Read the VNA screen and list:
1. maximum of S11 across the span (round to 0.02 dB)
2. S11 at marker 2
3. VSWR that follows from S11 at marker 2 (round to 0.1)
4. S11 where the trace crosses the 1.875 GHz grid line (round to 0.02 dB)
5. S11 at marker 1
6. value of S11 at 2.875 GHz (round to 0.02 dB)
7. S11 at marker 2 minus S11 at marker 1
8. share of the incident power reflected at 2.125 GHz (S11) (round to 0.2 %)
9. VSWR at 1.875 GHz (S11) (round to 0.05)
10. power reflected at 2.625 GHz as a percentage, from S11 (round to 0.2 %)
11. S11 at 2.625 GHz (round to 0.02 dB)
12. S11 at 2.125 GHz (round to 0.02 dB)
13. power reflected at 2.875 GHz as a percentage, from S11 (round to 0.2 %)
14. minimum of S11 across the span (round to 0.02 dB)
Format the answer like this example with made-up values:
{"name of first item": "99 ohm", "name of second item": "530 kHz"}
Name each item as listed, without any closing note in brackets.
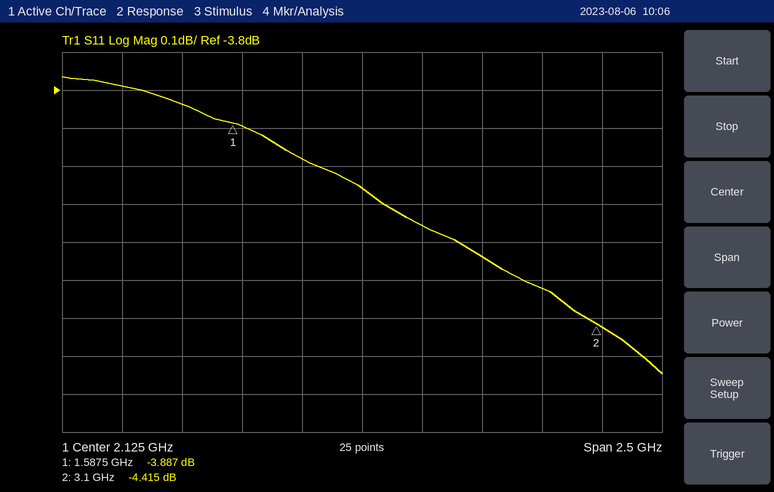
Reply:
{"maximum of S11 across the span": "-3.76 dB", "S11 at marker 2": "-4.415 dB", "VSWR that follows from S11 at marker 2": "4.0", "S11 where the trace crosses the 1.875 GHz grid line": "-3.98 dB", "S11 at marker 1": "-3.887 dB", "value of S11 at 2.875 GHz": "-4.32 dB", "S11 at marker 2 minus S11 at marker 1": "-0.528 dB", "share of the incident power reflected at 2.125 GHz (S11)": "39.2 %", "VSWR at 1.875 GHz (S11)": "4.45", "power reflected at 2.625 GHz as a percentage, from S11": "37.6 %", "S11 at 2.625 GHz": "-4.24 dB", "S11 at 2.125 GHz": "-4.06 dB", "power reflected at 2.875 GHz as a percentage, from S11": "37.0 %", "minimum of S11 across the span": "-4.54 dB"}
